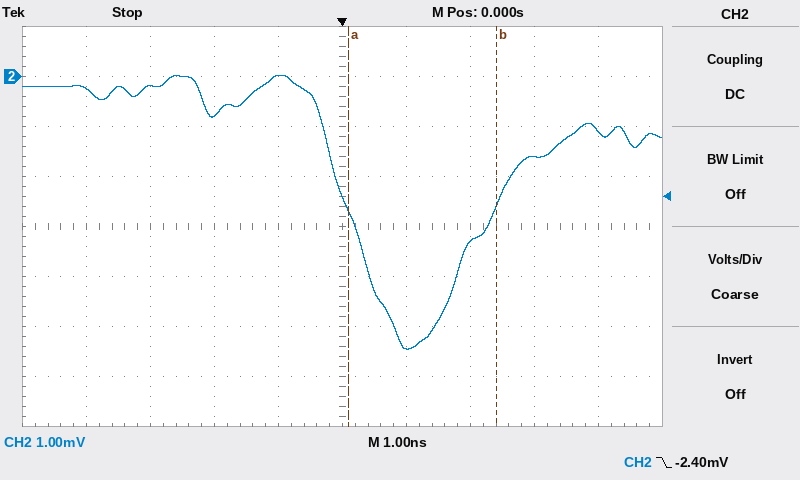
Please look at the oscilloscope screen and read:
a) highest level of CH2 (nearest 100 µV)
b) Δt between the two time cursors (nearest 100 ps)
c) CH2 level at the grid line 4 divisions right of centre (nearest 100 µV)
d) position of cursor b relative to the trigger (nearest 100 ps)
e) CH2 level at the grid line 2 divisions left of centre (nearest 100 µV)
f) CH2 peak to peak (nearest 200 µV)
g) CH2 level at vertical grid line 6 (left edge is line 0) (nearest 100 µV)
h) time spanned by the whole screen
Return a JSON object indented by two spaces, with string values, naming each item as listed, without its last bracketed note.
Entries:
{
  "highest level of CH2": "0.0 mV",
  "Δt between the two time cursors": "2.3 ns",
  "CH2 level at the grid line 4 divisions right of centre": "-1.1 mV",
  "position of cursor b relative to the trigger": "+2.4 ns",
  "CH2 level at the grid line 2 divisions left of centre": "-800 µV",
  "CH2 peak to peak": "5.4 mV",
  "CH2 level at vertical grid line 6 (left edge is line 0)": "-5.4 mV",
  "time spanned by the whole screen": "10 ns"
}
